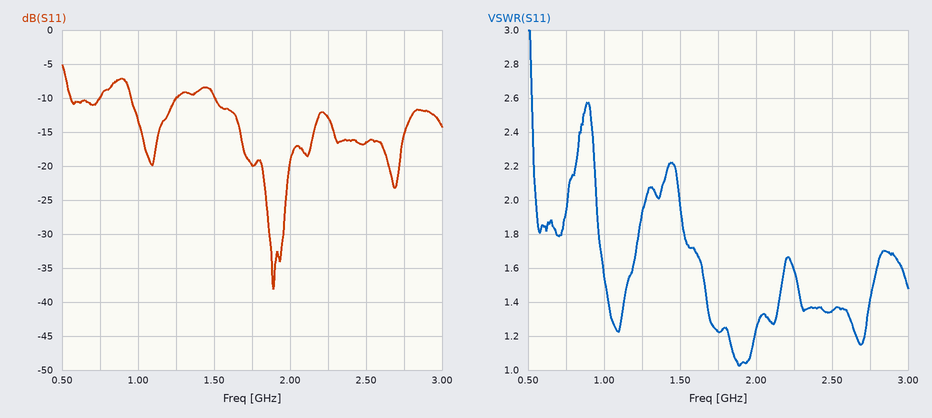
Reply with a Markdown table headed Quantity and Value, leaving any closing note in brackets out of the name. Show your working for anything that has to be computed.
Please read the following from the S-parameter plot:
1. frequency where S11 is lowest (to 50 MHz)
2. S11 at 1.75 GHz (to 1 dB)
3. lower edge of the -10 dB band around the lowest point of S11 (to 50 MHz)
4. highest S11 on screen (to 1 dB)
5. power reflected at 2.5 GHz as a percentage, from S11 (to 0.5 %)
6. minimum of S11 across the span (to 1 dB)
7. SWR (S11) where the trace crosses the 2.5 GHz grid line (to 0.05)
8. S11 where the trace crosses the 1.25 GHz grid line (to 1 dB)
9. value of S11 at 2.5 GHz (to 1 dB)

| Quantity | Value |
|---|---|
| frequency where S11 is lowest | 1.90 GHz |
| S11 at 1.75 GHz | -20 dB |
| lower edge of the -10 dB band around the lowest point of S11 | 1.50 GHz |
| highest S11 on screen | -5 dB |
| power reflected at 2.5 GHz as a percentage, from S11 | 10^(-17/10) ≈ 2.0 % |
| minimum of S11 across the span | -38 dB |
| SWR (S11) where the trace crosses the 2.5 GHz grid line | 1.35 |
| S11 where the trace crosses the 1.25 GHz grid line | -10 dB |
| value of S11 at 2.5 GHz | -17 dB |
